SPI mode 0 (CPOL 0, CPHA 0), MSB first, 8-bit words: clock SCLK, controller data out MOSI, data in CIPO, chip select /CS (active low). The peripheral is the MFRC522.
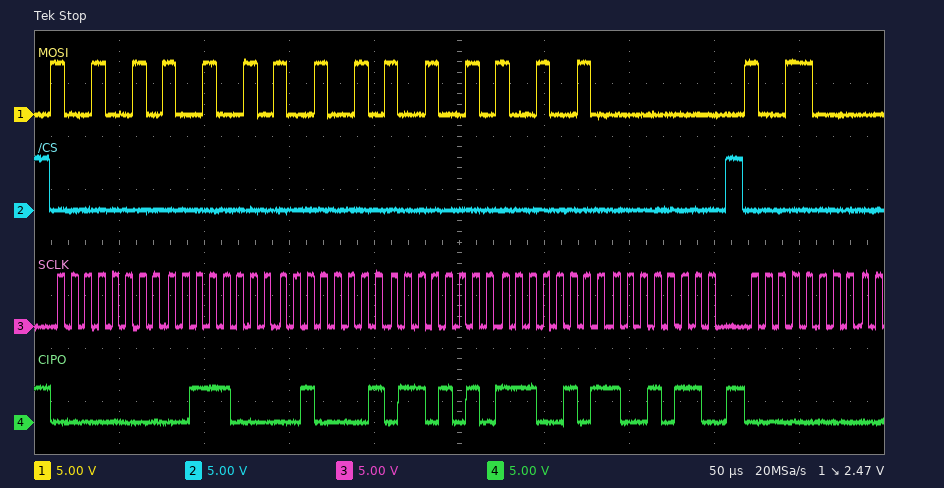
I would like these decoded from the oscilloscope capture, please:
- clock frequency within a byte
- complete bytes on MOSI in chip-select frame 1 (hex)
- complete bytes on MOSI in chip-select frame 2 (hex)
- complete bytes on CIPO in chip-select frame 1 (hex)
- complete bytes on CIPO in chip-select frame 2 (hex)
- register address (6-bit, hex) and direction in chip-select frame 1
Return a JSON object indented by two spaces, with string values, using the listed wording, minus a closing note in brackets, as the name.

{
  "clock frequency within a byte": "125 kHz",
  "complete bytes on MOSI in chip-select frame 1": "0x92 0x92 0x92 0x92 0x92 0x00",
  "complete bytes on MOSI in chip-select frame 2": "0x98",
  "complete bytes on CIPO in chip-select frame 1": "0x00 0x38 0x21 0x6A 0xE5 0x96",
  "complete bytes on CIPO in chip-select frame 2": "0x00",
  "register address (6-bit, hex) and direction in chip-select frame 1": "0x09 read"
}
